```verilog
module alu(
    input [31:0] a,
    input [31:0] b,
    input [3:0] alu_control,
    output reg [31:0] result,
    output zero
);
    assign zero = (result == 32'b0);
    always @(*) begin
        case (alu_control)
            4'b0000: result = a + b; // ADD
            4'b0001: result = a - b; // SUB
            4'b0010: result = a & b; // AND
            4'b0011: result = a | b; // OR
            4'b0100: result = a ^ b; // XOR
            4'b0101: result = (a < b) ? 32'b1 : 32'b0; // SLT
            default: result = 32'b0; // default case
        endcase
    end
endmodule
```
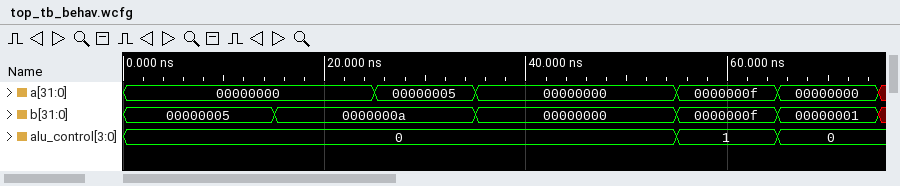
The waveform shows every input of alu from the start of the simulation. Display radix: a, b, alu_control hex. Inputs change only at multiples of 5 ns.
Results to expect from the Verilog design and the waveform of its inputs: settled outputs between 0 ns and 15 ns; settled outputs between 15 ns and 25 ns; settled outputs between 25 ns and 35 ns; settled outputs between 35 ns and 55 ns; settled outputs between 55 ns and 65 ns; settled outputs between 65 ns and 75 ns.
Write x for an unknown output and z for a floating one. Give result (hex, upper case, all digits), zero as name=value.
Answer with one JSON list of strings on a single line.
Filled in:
["result=00000005, zero=0", "result=0000000A, zero=0", "result=0000000F, zero=0", "result=00000000, zero=1", "result=00000000, zero=1", "result=00000001, zero=0"]
